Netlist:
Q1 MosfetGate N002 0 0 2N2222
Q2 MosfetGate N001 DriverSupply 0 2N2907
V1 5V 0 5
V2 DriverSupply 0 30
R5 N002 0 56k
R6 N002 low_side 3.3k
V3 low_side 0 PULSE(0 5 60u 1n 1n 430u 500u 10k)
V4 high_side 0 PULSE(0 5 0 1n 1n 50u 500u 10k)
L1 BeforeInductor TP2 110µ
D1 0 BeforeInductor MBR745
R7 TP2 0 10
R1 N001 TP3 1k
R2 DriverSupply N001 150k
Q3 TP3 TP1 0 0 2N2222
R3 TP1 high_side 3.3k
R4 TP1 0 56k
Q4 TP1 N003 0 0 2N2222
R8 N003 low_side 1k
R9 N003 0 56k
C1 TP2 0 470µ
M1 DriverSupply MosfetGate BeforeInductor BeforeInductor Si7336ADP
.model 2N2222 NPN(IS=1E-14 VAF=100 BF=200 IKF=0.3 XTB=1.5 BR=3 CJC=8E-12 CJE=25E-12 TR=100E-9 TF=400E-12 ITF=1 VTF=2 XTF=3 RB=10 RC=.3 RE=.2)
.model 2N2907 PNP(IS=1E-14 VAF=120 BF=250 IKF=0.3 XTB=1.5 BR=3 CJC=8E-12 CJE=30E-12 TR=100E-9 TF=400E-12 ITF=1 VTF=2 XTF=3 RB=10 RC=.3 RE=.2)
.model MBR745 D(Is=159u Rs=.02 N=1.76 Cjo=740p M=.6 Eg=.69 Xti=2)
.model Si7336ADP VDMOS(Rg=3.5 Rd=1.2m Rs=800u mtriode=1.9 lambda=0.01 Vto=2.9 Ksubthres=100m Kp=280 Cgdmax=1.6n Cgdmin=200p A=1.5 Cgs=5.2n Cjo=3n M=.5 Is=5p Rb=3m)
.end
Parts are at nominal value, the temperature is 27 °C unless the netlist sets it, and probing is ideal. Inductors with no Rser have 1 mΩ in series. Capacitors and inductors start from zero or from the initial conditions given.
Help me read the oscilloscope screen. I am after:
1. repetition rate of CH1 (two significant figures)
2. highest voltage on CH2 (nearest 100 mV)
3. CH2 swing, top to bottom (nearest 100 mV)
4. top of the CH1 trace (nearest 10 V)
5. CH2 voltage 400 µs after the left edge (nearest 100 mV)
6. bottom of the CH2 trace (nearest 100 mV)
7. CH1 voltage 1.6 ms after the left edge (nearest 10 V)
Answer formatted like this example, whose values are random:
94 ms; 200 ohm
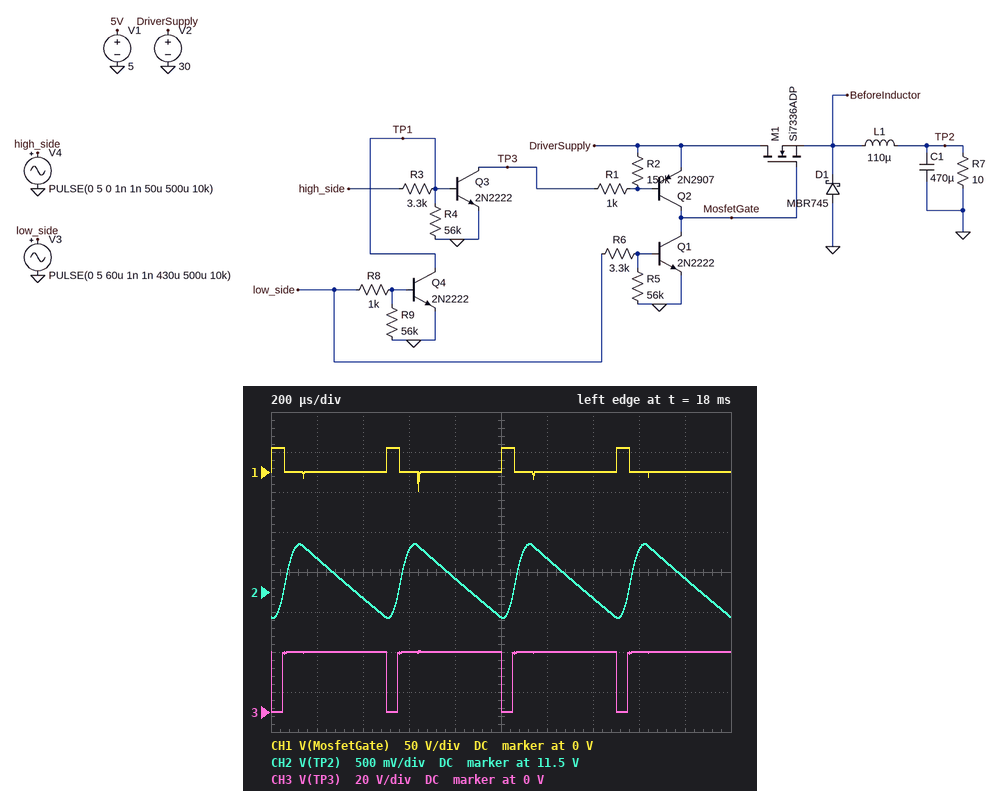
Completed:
2.0 kHz; 12.1 V; 900 mV; 30 V; 11.4 V; 11.2 V; 0 V
